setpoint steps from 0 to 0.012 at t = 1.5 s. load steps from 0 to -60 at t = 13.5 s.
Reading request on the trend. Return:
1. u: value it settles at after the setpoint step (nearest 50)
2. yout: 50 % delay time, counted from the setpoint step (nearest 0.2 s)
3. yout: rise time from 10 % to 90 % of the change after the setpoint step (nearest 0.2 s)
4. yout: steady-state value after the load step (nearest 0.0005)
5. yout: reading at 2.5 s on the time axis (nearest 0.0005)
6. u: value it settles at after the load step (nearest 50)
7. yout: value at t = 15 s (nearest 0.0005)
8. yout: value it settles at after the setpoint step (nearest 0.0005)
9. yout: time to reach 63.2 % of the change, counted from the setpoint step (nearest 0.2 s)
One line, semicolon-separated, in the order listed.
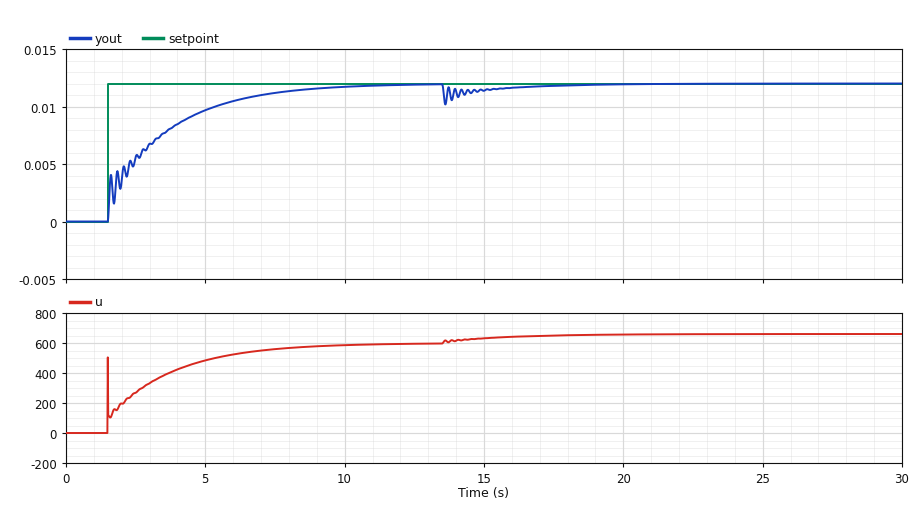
600; 1.2 s; 5.0 s; 0.0120; 0.0055; 650; 0.0115; 0.0120; 2.0 s
